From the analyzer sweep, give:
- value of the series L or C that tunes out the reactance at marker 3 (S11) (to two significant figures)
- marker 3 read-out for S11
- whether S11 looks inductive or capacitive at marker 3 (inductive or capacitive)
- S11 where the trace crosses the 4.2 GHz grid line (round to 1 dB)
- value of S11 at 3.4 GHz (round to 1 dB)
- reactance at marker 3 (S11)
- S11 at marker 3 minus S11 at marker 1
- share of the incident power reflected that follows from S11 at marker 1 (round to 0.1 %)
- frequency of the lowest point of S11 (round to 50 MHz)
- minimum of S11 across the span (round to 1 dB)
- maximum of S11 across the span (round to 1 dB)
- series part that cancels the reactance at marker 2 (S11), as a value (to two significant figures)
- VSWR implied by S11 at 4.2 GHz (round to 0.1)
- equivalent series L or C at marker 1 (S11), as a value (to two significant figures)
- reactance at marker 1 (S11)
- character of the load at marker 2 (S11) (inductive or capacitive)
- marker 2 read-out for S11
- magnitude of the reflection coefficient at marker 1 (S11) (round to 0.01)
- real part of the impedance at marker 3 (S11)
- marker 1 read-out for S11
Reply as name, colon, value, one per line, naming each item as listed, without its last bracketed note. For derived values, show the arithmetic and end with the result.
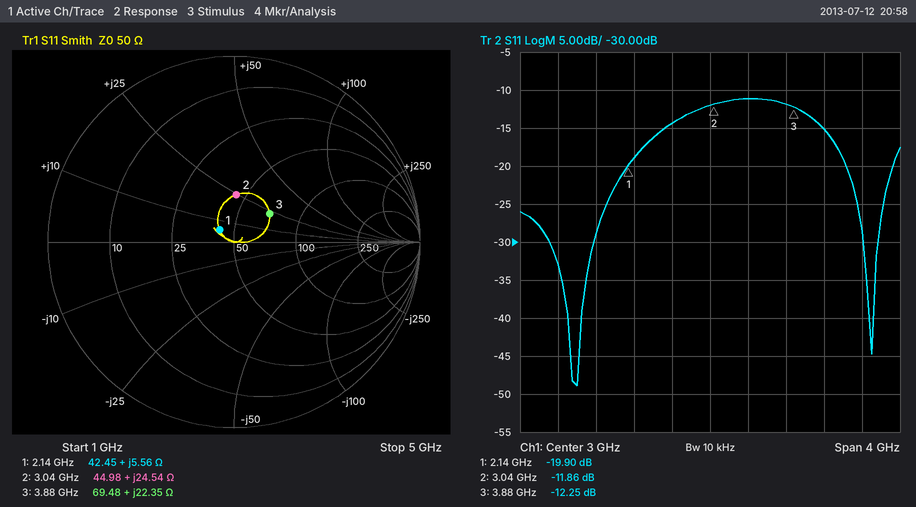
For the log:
value of the series L or C that tunes out the reactance at marker 3 (S11): C = 1/(2π × 3.88 GHz × 22.35 Ω) ≈ 1.8 pF
marker 3 read-out for S11: -12.25 dB
whether S11 looks inductive or capacitive at marker 3: inductive
S11 where the trace crosses the 4.2 GHz grid line: -15 dB
value of S11 at 3.4 GHz: -11 dB
reactance at marker 3: +22.35 Ω
S11 at marker 3 minus S11 at marker 1: -12.25 − (-19.9) = 7.65 dB
share of the incident power reflected that follows from S11 at marker 1: 10^(-19.9/10) ≈ 1.0 %
frequency of the lowest point of S11: 1.60 GHz
minimum of S11 across the span: -49 dB
maximum of S11 across the span: -11 dB
series part that cancels the reactance at marker 2 (S11), as a value: C = 1/(2π × 3.04 GHz × 24.54 Ω) ≈ 2.1 pF
VSWR implied by S11 at 4.2 GHz: |Γ| = 10^(-15/20) = 0.1778; VSWR = (1 + 0.1778)/(1 − 0.1778) ≈ 1.4
equivalent series L or C at marker 1 (S11), as a value: L = 5.56 Ω/(2π × 2.14 GHz) ≈ 414 pH, so 410 pH to two significant figures
reactance at marker 1: +5.56 Ω
character of the load at marker 2 (S11): inductive
marker 2 read-out for S11: -11.86 dB
magnitude of the reflection coefficient at marker 1 (S11): 0.10
real part of the impedance at marker 3: 69.48 Ω
marker 1 read-out for S11: -19.90 dB
